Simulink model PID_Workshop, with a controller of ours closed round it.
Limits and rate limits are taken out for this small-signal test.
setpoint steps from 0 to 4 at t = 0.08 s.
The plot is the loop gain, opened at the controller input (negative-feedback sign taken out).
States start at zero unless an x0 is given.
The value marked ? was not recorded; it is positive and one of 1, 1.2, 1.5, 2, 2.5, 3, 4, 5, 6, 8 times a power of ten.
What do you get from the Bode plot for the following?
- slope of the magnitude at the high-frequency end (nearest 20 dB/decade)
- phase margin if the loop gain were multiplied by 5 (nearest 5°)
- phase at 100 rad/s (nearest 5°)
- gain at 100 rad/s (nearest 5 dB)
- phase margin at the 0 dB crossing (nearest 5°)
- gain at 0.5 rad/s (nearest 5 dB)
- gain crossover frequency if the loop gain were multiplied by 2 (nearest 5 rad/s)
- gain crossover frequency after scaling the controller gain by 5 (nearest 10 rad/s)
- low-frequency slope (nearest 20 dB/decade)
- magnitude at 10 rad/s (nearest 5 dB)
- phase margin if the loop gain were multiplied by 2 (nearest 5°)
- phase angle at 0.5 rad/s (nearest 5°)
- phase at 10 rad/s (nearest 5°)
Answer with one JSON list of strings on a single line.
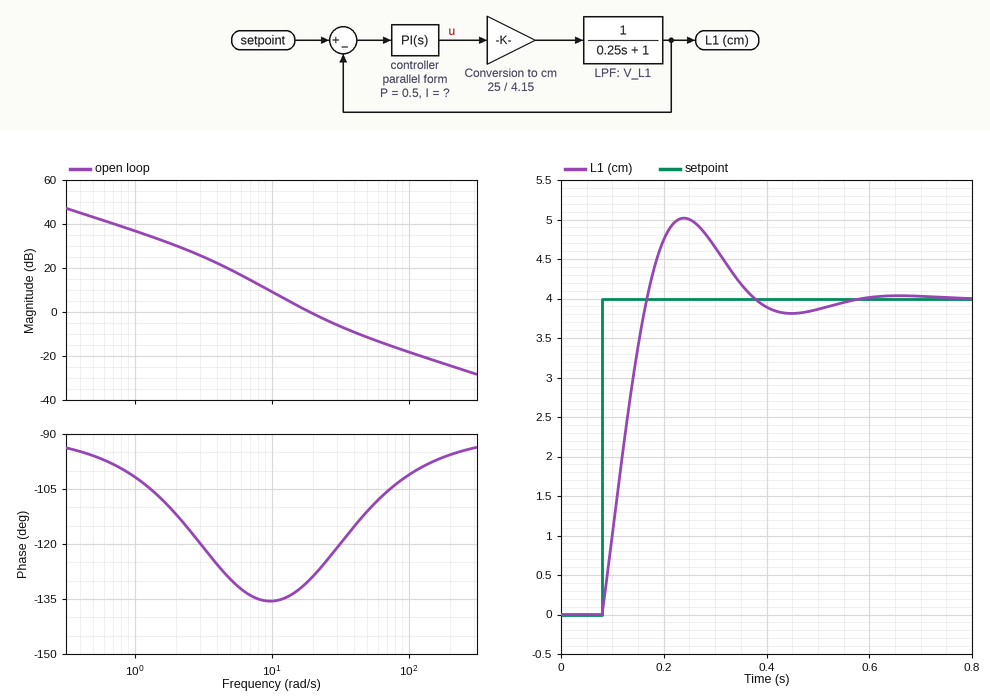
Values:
["-20 dB/decade", "75°", "-100°", "-20 dB", "50°", "45 dB", "30 rad/s", "60 rad/s", "-20 dB/decade", "10 dB", "60°", "-95°", "-135°"]
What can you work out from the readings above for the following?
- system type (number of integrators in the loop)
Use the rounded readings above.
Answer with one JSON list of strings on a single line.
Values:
["1"]
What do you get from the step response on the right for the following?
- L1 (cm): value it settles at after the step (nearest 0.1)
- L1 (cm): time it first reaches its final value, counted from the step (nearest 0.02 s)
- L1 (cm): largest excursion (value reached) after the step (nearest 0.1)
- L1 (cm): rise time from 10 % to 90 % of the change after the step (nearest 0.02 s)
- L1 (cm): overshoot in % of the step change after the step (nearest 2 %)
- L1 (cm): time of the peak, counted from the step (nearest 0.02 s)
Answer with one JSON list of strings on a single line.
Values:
["4.0", "0.08 s", "5.0", "0.06 s", "26 %", "0.16 s"]
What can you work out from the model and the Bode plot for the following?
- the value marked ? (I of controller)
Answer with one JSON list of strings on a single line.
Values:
["12"]
